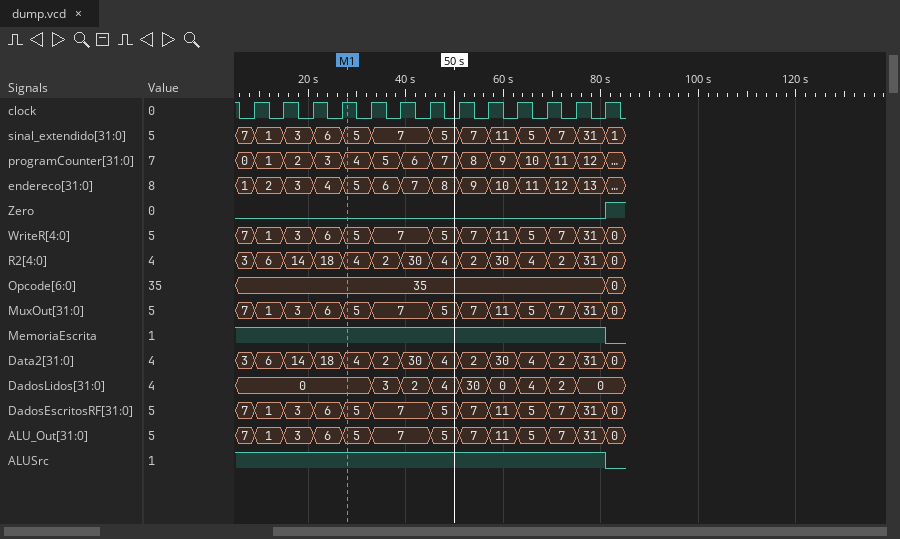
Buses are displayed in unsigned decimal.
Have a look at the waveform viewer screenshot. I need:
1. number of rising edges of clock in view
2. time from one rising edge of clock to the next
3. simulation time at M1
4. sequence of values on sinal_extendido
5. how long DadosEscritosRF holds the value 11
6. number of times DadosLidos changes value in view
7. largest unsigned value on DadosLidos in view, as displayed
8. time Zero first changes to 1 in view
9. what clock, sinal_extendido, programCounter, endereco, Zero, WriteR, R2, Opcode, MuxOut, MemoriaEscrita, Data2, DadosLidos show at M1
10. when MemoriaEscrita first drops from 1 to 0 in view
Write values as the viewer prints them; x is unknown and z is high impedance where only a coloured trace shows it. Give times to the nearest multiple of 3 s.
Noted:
13
6 s
27 s
7, 1, 3, 6, 5, 7, 5, 7, 11, 5, 7, 31, 1
6 s
8
30
81 s
clock=1, sinal_extendido=5, programCounter=4, endereco=5, Zero=0, WriteR=5, R2=4, Opcode=35, MuxOut=5, MemoriaEscrita=1, Data2=4, DadosLidos=0
81 s
